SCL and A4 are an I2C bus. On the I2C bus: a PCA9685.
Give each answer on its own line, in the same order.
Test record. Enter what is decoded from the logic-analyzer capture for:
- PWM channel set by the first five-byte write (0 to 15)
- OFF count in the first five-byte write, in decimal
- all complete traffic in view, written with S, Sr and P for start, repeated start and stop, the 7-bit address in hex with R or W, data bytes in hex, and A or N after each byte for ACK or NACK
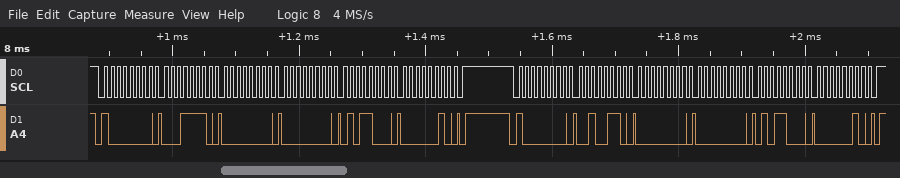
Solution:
6
600
S 40W A 1E A 00 A 00 A 58 A 02 A P S 40W A 26 A 00 A 00 A 58 A 02 A P
